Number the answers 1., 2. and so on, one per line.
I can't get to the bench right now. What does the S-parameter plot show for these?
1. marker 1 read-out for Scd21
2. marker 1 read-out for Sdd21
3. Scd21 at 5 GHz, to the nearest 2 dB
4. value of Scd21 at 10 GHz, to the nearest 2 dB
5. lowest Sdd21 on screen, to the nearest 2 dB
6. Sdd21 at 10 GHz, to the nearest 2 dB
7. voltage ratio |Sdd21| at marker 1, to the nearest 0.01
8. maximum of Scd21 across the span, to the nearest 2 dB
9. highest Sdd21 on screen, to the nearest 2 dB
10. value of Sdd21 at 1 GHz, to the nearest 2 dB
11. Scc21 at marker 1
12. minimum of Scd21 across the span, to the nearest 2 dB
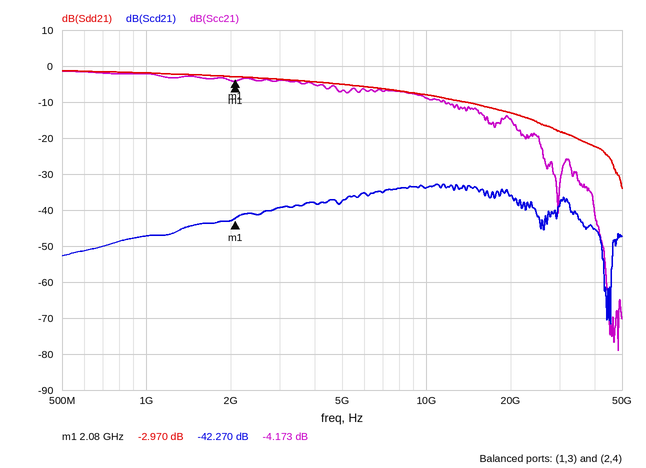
1. -42.270 dB
2. -2.970 dB
3. -38 dB
4. -34 dB
5. -34 dB
6. -8 dB
7. 0.71
8. -32 dB
9. -2 dB
10. -2 dB
11. -4.173 dB
12. -72 dB
